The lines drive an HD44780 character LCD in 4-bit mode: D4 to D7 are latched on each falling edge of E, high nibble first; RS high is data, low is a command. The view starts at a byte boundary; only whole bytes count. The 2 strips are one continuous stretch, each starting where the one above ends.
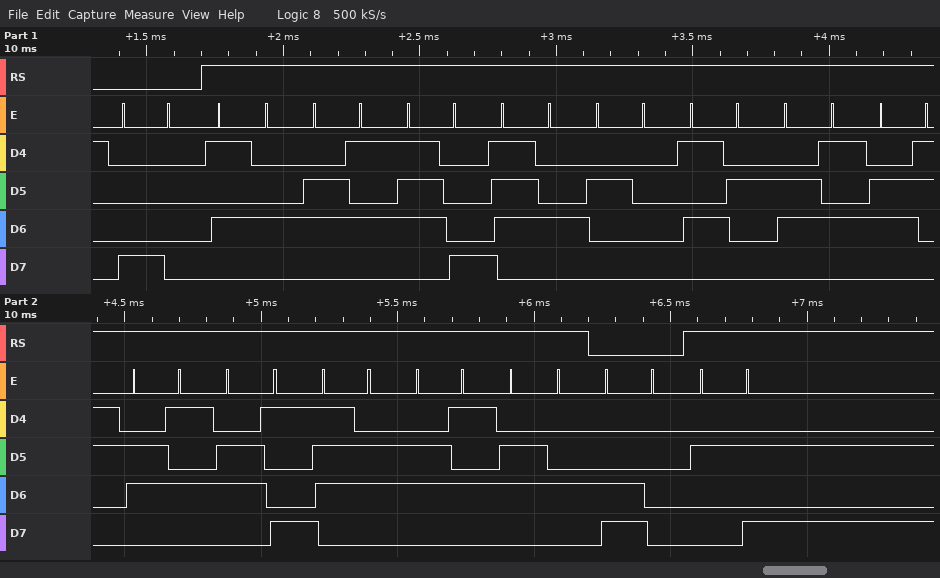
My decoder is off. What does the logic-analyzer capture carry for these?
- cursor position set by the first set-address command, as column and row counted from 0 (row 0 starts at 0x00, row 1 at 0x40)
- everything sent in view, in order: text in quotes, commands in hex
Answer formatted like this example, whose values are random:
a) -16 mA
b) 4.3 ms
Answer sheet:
a) column 0, row 0
b) 0x80 "Text Received" 0xC0 "*"
